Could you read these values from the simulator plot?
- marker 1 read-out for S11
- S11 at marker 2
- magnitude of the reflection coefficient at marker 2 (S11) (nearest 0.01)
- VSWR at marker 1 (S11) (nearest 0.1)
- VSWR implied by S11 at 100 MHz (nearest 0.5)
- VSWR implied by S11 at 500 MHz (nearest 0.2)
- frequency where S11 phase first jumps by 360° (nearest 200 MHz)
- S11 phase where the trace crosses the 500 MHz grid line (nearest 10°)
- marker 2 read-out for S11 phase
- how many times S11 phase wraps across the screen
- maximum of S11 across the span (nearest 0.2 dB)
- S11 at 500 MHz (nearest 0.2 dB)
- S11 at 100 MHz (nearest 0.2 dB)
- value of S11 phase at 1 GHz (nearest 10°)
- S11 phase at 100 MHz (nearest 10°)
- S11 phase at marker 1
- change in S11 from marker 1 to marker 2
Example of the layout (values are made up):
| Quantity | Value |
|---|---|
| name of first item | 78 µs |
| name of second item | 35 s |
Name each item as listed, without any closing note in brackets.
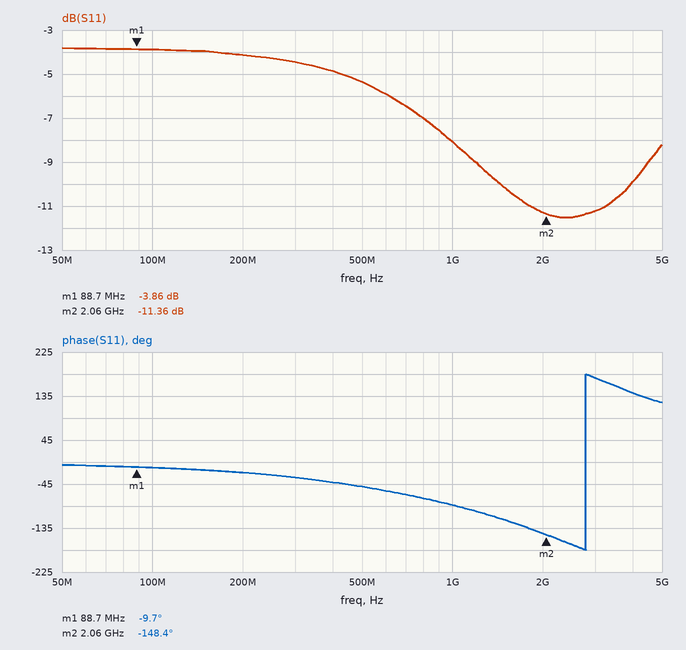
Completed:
| Quantity | Value |
|---|---|
| marker 1 read-out for S11 | -3.86 dB |
| S11 at marker 2 | -11.36 dB |
| magnitude of the reflection coefficient at marker 2 (S11) | 0.27 |
| VSWR at marker 1 (S11) | 4.6 |
| VSWR implied by S11 at 100 MHz | 4.5 |
| VSWR implied by S11 at 500 MHz | 3.4 |
| frequency where S11 phase first jumps by 360° | 2.8 GHz |
| S11 phase where the trace crosses the 500 MHz grid line | -50° |
| marker 2 read-out for S11 phase | -148.4° |
| how many times S11 phase wraps across the screen | 1 |
| maximum of S11 across the span | -3.8 dB |
| S11 at 500 MHz | -5.4 dB |
| S11 at 100 MHz | -3.8 dB |
| value of S11 phase at 1 GHz | -90° |
| S11 phase at 100 MHz | -10° |
| S11 phase at marker 1 | -9.7° |
| change in S11 from marker 1 to marker 2 | -7.50 dB |
